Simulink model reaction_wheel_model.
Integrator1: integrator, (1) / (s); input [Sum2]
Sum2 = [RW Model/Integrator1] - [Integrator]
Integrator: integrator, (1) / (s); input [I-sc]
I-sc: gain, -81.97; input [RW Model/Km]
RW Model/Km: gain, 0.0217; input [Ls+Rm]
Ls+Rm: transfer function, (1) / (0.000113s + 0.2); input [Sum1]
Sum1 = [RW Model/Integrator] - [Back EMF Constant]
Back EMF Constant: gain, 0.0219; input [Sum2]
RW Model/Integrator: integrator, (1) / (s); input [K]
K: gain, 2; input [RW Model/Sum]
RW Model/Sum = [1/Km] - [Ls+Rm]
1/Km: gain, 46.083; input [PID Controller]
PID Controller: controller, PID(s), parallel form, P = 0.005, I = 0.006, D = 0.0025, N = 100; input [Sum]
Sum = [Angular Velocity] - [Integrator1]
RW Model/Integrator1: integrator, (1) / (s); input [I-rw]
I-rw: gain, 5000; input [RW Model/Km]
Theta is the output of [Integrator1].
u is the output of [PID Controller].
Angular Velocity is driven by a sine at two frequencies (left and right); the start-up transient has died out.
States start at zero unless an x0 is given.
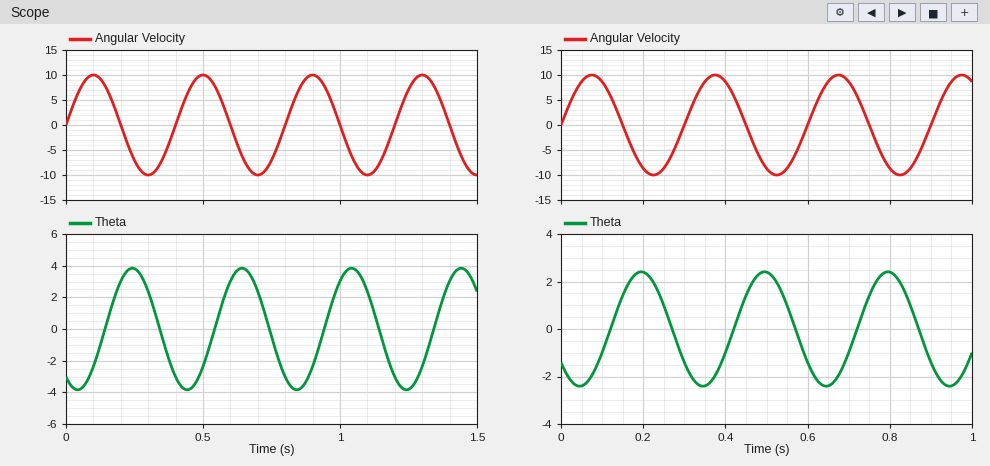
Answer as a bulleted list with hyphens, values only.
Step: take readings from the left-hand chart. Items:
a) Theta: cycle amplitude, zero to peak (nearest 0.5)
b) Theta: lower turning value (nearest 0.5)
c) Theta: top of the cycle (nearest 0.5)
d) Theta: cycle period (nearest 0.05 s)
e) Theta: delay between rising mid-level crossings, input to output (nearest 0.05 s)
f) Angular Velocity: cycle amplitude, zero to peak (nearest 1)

- 4.0
- -4.0
- 4.0
- 0.40 s
- 0.15 s
- 10
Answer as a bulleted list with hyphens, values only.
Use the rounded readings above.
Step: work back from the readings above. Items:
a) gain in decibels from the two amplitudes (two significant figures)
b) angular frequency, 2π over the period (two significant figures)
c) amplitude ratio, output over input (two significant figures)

- -8.0 dB
- 16 rad/s
- 0.40
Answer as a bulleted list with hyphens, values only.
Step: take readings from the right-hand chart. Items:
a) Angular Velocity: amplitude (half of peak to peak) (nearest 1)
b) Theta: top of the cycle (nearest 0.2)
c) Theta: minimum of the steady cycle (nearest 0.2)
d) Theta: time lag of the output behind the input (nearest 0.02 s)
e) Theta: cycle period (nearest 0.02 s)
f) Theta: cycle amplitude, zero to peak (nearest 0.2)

- 10
- 2.4
- -2.4
- 0.12 s
- 0.30 s
- 2.4
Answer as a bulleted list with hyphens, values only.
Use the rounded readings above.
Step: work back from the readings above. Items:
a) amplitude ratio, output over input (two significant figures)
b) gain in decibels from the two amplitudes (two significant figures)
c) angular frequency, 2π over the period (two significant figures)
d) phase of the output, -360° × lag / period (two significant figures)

- 0.24
- -12 dB
- 21 rad/s
- -140°
